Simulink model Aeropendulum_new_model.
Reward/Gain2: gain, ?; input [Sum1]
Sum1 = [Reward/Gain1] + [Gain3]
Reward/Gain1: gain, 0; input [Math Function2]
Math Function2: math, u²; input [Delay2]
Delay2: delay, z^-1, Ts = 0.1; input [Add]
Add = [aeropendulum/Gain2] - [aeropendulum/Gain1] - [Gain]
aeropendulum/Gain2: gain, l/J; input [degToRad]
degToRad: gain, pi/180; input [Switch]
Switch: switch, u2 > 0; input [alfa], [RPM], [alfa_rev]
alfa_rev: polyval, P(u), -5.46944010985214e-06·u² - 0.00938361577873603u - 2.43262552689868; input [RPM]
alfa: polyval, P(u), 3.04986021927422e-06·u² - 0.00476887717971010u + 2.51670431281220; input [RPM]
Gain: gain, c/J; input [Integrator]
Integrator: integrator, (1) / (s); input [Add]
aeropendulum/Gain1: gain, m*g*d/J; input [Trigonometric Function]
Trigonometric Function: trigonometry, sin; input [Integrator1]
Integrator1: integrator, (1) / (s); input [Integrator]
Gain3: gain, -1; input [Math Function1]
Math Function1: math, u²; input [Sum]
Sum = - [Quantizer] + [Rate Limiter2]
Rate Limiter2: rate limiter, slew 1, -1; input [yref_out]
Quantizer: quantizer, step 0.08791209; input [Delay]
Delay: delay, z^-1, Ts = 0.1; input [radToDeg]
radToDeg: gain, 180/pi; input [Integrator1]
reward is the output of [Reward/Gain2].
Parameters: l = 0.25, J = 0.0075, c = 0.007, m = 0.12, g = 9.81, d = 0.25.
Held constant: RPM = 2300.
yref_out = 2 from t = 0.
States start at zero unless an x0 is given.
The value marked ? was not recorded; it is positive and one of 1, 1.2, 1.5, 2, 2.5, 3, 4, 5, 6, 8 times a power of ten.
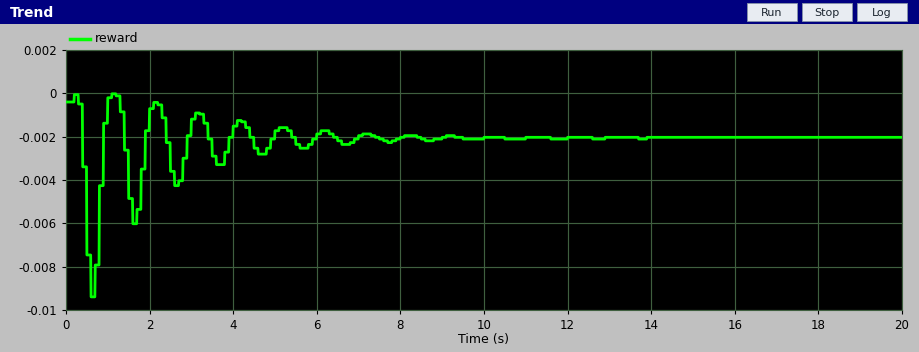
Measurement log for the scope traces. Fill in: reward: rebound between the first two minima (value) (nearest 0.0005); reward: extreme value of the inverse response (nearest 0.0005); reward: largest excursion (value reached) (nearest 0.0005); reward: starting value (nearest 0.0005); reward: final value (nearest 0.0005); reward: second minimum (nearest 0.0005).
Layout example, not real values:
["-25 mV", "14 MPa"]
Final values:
["0.0000", "0.0000", "-0.0095", "-0.0005", "-0.0020", "-0.0060"]
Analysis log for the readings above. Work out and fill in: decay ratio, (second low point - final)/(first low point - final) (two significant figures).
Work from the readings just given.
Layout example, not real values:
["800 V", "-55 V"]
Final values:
["0.53"]
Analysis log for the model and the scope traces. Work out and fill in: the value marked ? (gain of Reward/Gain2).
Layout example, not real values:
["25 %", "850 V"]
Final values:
["0.0001"]
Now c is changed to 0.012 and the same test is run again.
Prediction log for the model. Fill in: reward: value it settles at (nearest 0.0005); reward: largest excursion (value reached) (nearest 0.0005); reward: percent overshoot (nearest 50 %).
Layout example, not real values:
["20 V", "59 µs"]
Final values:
["-0.0020", "-0.0080", "350 %"]
